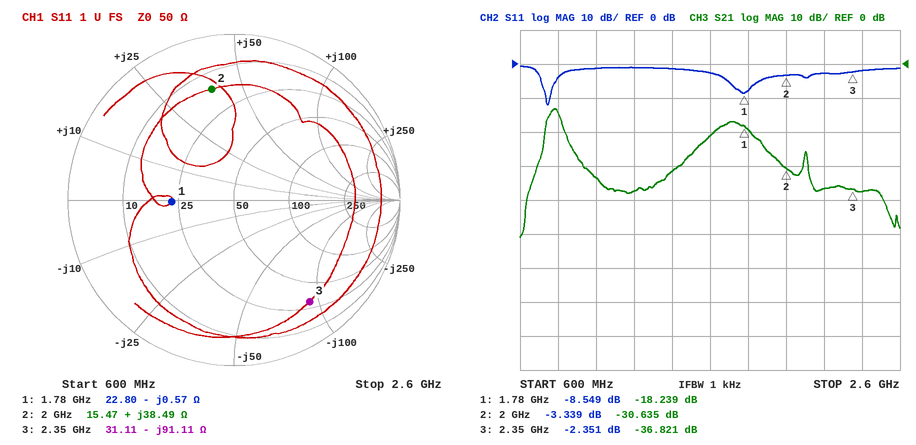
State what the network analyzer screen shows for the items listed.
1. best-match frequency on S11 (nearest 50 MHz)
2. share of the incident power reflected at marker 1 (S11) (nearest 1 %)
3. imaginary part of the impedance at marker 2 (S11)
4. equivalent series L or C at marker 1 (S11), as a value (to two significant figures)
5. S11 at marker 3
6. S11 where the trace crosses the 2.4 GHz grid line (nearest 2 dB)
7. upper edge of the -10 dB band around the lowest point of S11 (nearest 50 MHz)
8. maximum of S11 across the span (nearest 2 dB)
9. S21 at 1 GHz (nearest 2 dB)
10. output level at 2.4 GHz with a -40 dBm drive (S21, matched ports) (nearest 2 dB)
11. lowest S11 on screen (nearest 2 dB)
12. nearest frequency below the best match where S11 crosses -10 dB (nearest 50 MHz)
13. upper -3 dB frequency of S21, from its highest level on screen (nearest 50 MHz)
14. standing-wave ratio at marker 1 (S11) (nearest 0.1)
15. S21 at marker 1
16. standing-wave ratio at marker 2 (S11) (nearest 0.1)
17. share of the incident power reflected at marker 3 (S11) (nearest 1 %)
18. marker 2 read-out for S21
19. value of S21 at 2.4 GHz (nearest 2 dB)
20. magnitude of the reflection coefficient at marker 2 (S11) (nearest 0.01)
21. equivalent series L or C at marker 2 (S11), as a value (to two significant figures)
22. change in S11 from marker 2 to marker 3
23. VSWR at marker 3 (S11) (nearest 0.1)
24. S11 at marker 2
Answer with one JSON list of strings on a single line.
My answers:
["750 MHz", "14 %", "+38.49 Ω", "160 pF", "-2.351 dB", "-2 dB", "750 MHz", "0 dB", "-34 dB", "-78 dBm", "-12 dB", "750 MHz", "800 MHz", "2.2", "-18.239 dB", "5.3", "58 %", "-30.635 dB", "-38 dB", "0.68", "3.1 nH", "0.988 dB", "7.4", "-3.339 dB"]
